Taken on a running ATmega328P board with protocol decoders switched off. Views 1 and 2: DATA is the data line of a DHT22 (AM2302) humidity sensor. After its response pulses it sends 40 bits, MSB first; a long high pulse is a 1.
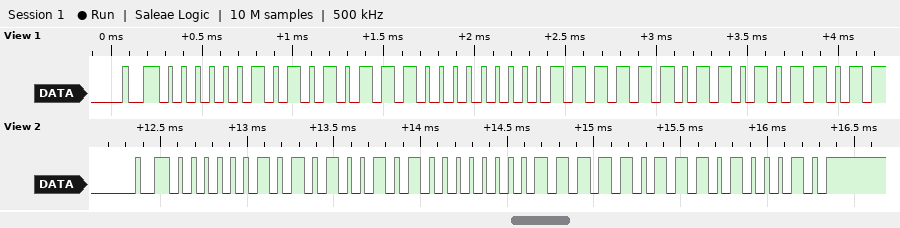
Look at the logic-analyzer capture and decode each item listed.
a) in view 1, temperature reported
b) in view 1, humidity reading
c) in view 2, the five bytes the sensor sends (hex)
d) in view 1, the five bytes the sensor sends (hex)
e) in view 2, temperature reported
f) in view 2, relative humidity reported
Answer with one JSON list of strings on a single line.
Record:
["25.3 °C", "68.6 %", "02 A5 00 FB A2", "02 AE 00 FD AD", "25.1 °C", "67.7 %"]
